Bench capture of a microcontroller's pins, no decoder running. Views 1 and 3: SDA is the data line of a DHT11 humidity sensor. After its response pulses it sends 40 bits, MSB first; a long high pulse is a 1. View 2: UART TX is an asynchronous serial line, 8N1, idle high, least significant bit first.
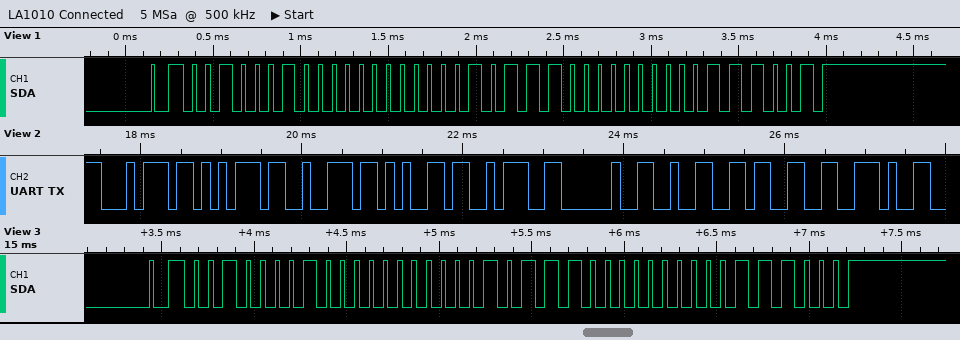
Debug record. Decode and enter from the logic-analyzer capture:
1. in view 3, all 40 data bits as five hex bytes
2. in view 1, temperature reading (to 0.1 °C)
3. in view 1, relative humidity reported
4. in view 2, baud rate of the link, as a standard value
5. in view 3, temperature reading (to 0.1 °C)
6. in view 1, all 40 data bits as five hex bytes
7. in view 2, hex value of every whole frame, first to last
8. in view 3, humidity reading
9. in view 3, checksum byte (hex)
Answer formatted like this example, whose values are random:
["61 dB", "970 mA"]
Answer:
["21 00 17 00 38", "23.0 °C", "34 %", "9600 baud", "23.0 °C", "22 00 17 00 39", "0x74 0x75 0x72 0x65 0x3A 0x20 0x32 0x33 0x2E", "33 %", "0x38"]
